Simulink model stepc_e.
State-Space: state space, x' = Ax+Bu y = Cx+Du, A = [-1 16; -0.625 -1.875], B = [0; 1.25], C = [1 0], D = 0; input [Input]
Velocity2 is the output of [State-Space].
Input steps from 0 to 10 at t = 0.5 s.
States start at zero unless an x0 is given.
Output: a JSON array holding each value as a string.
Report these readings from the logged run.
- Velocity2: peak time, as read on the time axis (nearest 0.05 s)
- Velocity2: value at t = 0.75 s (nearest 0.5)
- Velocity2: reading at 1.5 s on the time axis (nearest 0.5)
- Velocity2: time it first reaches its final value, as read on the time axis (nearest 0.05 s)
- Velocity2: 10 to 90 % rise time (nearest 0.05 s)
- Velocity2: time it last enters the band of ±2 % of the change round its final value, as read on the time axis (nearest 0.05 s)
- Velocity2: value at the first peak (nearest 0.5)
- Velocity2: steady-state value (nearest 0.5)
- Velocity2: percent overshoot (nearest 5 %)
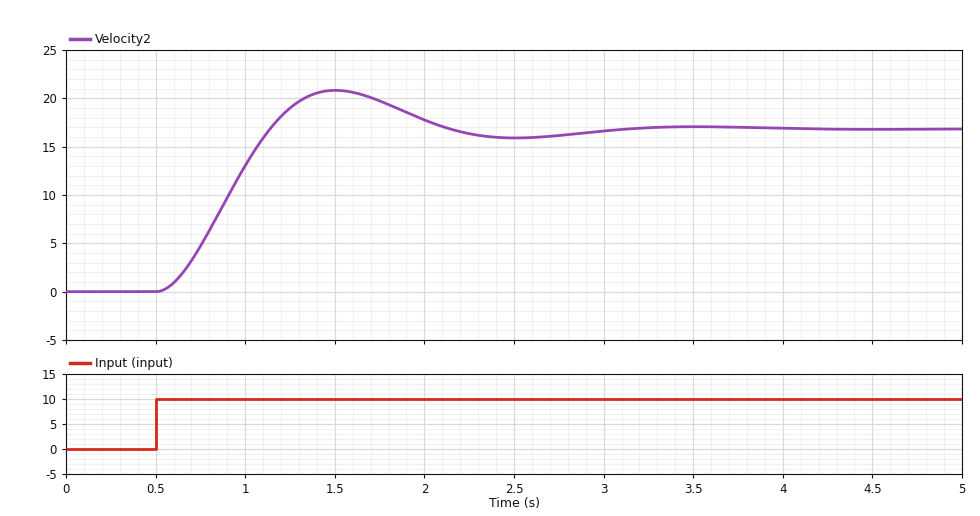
["1.50 s", "4.5", "21.0", "1.15 s", "0.45 s", "2.95 s", "21.0", "17.0", "25 %"]
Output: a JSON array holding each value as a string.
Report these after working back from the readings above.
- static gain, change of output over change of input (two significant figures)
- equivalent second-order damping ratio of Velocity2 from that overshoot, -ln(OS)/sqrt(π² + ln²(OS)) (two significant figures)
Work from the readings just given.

["1.7", "0.40"]
